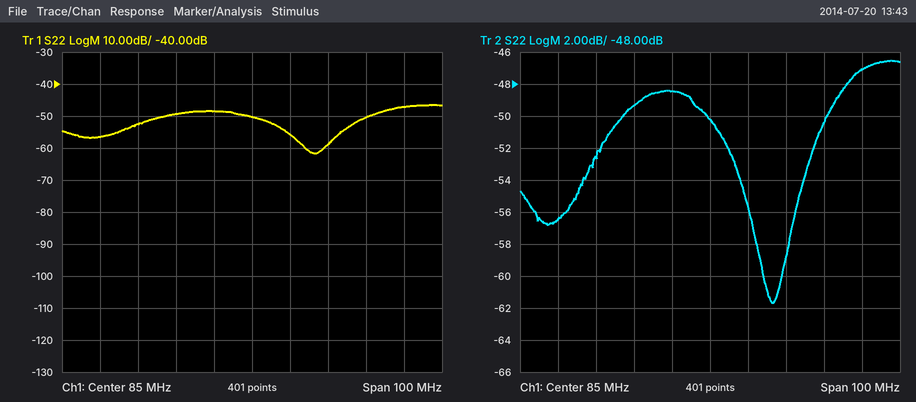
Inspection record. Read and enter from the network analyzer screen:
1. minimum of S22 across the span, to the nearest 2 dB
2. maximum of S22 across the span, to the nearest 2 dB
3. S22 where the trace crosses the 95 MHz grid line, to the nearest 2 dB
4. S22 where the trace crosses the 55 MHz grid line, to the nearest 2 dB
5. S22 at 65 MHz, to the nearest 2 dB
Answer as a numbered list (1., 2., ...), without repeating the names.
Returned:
1. -62 dB
2. -46 dB
3. -56 dB
4. -52 dB
5. -50 dB
